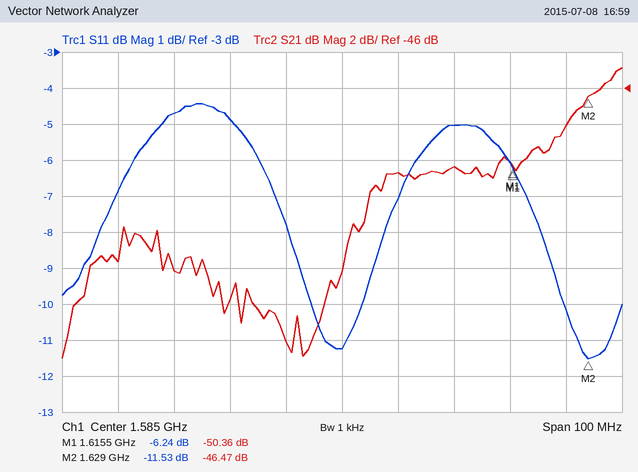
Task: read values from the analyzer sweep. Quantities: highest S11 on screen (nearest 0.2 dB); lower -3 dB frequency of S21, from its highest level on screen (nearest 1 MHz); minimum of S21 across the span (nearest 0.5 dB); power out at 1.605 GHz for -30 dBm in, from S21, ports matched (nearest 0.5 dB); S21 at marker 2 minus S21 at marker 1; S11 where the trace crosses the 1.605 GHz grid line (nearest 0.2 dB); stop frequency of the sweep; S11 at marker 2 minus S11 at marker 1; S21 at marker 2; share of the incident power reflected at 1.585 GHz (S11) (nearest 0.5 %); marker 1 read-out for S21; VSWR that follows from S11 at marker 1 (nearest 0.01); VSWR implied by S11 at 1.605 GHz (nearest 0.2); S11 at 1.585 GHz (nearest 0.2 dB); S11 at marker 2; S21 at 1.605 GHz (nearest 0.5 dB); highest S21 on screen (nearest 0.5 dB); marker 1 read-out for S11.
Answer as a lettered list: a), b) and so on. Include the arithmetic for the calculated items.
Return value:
a) -4.4 dB
b) 1.625 GHz
c) -61.0 dB
d) -30 dBm + (-50.5 dB) = -80.5 dBm
e) -46.47 − (-50.36) = 3.89 dB
f) -5.0 dB
g) 1.635 GHz
h) -11.53 − (-6.24) = -5.29 dB
i) -46.47 dB
j) 10^(-11.2/10) ≈ 7.59 %, so 7.5 % to the nearest 0.5 %
k) -50.36 dB
l) (1 + 0.4875)/(1 − 0.4875) ≈ 2.90
m) |Γ| = 10^(-5/20) = 0.5623; VSWR = (1 + 0.5623)/(1 − 0.5623) ≈ 3.6
n) -11.2 dB
o) -11.53 dB
p) -50.5 dB
q) -45.0 dB
r) -6.24 dB
